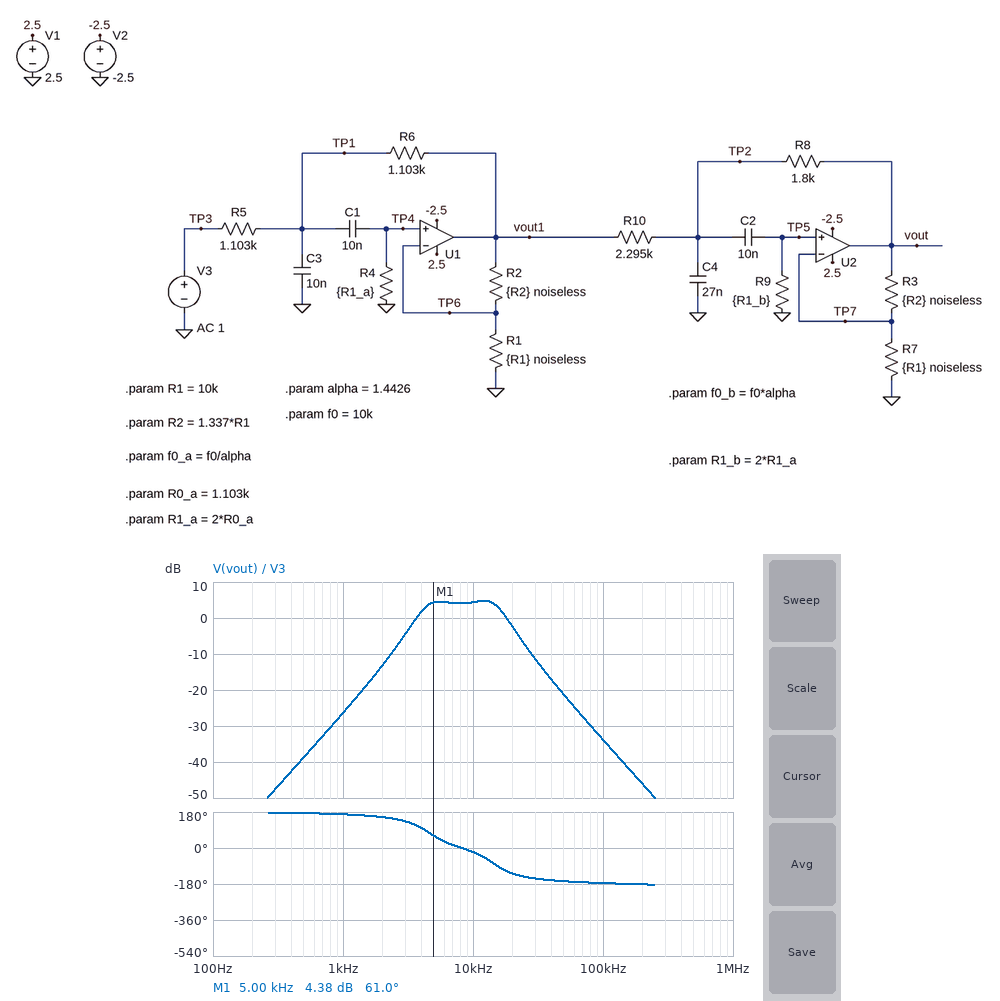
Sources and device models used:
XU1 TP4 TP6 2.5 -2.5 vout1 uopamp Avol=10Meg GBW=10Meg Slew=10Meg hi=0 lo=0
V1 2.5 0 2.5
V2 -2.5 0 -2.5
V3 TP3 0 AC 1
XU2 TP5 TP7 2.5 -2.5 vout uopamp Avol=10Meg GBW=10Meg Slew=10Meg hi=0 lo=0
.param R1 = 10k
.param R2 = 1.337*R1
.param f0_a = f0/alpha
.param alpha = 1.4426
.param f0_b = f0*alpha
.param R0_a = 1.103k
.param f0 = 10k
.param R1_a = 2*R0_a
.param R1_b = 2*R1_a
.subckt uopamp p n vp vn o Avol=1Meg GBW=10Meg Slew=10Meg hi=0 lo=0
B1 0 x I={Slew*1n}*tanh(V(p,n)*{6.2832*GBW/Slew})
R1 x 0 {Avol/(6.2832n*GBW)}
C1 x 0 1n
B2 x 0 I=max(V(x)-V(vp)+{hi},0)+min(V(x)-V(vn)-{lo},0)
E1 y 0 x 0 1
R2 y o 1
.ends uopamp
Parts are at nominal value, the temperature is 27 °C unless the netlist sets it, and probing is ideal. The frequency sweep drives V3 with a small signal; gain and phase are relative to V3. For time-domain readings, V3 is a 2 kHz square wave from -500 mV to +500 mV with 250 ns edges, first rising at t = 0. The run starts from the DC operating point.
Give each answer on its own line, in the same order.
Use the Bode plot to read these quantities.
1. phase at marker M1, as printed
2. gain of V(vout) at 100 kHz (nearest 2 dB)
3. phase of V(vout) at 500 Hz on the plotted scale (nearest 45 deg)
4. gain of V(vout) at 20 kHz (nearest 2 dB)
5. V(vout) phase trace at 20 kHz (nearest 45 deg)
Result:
61.0 deg
-34 dB
180 deg
-2 dB
-135 deg
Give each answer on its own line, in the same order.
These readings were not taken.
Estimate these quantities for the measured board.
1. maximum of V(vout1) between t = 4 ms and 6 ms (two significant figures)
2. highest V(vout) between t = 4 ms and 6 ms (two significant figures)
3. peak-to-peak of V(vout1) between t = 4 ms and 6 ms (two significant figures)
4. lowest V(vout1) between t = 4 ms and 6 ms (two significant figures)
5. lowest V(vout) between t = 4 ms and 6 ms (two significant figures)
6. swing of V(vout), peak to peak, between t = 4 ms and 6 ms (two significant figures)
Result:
1.5 V
830 mV
3.0 V
-1.5 V
-830 mV
1.7 V
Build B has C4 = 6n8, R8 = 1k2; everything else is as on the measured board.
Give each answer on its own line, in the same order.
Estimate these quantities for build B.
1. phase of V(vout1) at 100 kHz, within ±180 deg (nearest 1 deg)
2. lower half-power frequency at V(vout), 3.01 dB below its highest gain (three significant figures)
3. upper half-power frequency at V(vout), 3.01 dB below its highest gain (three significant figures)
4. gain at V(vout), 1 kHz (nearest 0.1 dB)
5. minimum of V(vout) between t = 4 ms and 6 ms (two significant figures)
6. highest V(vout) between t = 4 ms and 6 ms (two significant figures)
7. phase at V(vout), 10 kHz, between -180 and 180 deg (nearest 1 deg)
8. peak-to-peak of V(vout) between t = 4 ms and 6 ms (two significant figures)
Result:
-86 deg
9.28 kHz
16.0 kHz
-28.8 dB
-2.5 V
2.5 V
-137 deg
5.0 V
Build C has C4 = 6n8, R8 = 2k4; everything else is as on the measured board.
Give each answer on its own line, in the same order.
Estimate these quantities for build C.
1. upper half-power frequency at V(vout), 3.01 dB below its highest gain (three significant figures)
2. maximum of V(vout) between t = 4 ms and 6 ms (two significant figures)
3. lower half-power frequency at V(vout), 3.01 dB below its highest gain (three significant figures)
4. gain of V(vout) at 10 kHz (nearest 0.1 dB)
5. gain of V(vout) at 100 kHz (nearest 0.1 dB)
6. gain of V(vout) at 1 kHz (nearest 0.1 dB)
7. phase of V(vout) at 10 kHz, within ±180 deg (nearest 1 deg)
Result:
16.0 kHz
2.5 V
7.79 kHz
18.4 dB
-21.8 dB
-25.3 dB
23 deg
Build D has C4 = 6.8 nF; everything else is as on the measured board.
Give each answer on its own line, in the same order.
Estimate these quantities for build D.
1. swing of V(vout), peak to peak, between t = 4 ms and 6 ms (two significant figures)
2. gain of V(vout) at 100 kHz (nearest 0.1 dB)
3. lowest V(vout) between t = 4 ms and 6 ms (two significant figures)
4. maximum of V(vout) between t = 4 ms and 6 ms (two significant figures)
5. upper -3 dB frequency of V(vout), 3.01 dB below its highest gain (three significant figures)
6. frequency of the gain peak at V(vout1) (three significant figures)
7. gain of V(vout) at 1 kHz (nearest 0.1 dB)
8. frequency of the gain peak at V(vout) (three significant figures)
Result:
5.0 V
-21.8 dB
-2.5 V
2.5 V
10.4 kHz
14.4 kHz
-26.6 dB
9.25 kHz
